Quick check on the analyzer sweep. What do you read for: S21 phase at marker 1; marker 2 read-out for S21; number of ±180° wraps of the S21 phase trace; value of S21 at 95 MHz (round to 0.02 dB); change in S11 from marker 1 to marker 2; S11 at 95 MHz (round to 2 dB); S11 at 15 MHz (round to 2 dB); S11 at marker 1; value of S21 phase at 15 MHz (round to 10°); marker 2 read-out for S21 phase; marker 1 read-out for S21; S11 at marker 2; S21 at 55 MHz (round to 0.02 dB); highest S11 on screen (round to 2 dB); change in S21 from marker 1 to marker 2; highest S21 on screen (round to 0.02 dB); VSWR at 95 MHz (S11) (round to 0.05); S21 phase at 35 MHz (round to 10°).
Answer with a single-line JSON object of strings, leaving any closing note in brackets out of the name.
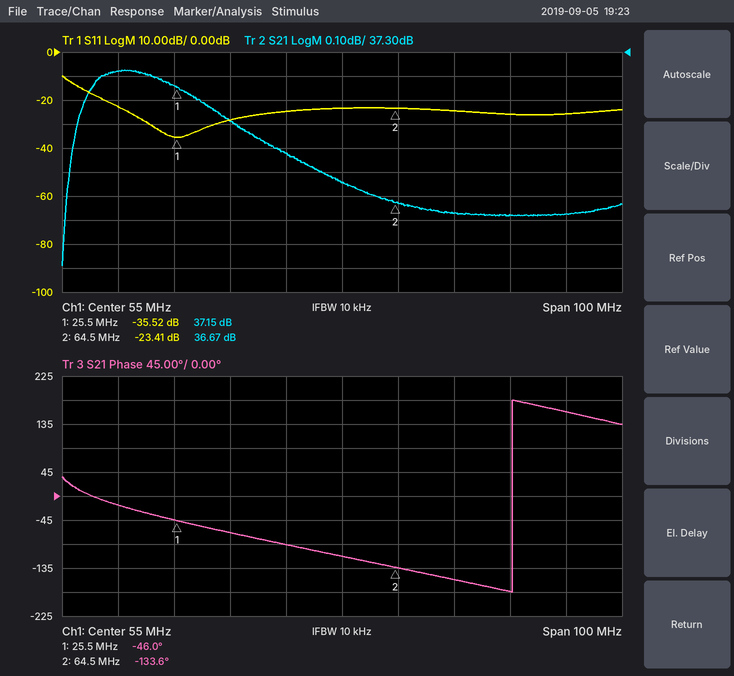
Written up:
{"S21 phase at marker 1": "-46.0°", "marker 2 read-out for S21": "36.67 dB", "number of ±180° wraps of the S21 phase trace": "1", "value of S21 at 95 MHz": "36.62 dB", "change in S11 from marker 1 to marker 2": "12.11 dB", "S11 at 95 MHz": "-26 dB", "S11 at 15 MHz": "-22 dB", "S11 at marker 1": "-35.52 dB", "value of S21 phase at 15 MHz": "-20°", "marker 2 read-out for S21 phase": "-133.6°", "marker 1 read-out for S21": "37.15 dB", "S11 at marker 2": "-23.41 dB", "S21 at 55 MHz": "36.76 dB", "highest S11 on screen": "-10 dB", "change in S21 from marker 1 to marker 2": "-0.48 dB", "highest S21 on screen": "37.22 dB", "VSWR at 95 MHz (S11)": "1.10", "S21 phase at 35 MHz": "-70°"}
